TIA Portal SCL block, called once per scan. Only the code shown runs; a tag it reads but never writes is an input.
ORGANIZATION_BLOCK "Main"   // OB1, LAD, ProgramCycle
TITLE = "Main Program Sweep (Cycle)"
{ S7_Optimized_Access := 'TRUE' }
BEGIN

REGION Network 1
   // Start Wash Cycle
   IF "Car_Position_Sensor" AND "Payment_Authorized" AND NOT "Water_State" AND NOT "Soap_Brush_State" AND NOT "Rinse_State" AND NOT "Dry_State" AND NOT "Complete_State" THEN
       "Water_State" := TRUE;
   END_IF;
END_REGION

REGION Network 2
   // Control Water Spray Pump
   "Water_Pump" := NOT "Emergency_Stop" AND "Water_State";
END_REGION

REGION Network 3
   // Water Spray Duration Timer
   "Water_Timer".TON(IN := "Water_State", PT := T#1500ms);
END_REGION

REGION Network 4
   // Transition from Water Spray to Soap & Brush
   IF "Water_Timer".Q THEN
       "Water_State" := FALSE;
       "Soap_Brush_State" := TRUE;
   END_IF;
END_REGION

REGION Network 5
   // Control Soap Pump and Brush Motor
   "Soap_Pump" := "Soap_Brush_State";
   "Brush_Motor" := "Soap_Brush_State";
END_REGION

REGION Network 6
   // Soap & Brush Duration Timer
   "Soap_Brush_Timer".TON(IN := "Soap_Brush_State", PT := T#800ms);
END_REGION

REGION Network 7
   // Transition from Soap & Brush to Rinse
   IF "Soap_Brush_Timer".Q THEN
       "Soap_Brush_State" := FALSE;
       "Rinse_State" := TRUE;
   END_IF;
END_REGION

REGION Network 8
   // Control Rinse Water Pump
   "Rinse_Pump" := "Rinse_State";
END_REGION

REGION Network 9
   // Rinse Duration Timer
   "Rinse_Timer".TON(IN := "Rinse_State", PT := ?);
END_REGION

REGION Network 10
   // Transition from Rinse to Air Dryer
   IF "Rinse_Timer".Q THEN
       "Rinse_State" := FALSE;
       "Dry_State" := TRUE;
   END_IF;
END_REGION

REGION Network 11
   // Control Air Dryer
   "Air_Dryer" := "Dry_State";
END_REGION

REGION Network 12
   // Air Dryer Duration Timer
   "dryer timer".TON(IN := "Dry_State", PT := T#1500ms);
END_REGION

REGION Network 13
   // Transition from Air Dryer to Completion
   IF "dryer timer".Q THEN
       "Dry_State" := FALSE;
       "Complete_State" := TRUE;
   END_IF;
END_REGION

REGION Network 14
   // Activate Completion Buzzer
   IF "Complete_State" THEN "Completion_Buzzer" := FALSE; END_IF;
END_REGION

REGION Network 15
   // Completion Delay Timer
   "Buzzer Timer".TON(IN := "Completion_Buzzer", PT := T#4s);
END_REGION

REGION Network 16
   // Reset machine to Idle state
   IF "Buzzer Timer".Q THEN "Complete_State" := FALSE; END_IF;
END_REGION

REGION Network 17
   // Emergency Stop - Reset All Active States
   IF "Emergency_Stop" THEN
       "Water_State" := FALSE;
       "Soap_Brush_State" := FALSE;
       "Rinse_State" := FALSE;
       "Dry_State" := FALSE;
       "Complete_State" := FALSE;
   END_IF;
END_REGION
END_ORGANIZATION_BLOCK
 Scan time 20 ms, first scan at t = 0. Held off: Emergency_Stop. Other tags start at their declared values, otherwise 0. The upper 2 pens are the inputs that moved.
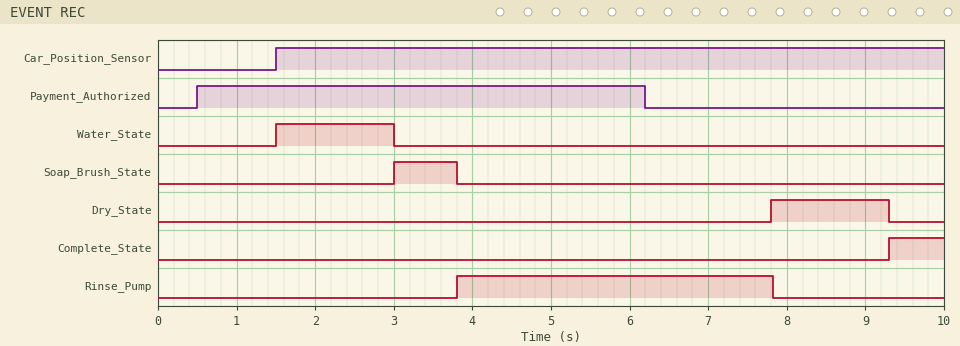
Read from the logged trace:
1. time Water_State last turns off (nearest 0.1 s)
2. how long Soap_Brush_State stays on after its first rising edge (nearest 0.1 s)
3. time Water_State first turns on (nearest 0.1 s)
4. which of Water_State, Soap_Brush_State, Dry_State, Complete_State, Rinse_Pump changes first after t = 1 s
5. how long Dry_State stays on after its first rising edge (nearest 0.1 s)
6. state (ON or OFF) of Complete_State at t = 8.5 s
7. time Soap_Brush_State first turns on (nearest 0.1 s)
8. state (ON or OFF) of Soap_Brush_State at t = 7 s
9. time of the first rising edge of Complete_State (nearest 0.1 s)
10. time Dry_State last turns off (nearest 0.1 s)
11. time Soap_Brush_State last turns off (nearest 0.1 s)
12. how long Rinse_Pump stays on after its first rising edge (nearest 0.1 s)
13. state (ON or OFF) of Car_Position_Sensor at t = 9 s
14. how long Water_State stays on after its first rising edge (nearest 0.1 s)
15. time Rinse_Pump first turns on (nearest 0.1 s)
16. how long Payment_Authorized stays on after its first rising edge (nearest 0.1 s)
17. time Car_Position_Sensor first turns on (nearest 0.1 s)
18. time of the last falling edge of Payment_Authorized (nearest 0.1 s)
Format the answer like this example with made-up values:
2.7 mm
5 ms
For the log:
3.0 s
0.8 s
1.5 s
Water_State
1.5 s
OFF
3.0 s
OFF
9.3 s
9.3 s
3.8 s
4.0 s
ON
1.5 s
3.8 s
5.7 s
1.5 s
6.2 s
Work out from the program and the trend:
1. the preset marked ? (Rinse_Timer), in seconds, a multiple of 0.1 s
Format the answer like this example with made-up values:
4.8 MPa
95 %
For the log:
4.0 s
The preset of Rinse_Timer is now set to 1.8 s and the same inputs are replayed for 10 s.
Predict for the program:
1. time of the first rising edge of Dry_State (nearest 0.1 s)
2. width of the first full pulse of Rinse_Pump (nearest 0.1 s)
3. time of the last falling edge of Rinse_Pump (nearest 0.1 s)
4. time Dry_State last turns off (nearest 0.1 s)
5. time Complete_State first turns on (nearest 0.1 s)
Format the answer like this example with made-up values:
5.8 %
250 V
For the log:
5.6 s
1.8 s
5.6 s
7.1 s
7.1 s
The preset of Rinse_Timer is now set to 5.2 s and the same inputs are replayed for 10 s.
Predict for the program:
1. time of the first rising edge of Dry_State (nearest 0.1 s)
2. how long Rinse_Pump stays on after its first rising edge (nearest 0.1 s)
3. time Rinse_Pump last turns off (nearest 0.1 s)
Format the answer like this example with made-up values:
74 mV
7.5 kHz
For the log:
9.0 s
5.2 s
9.0 s
